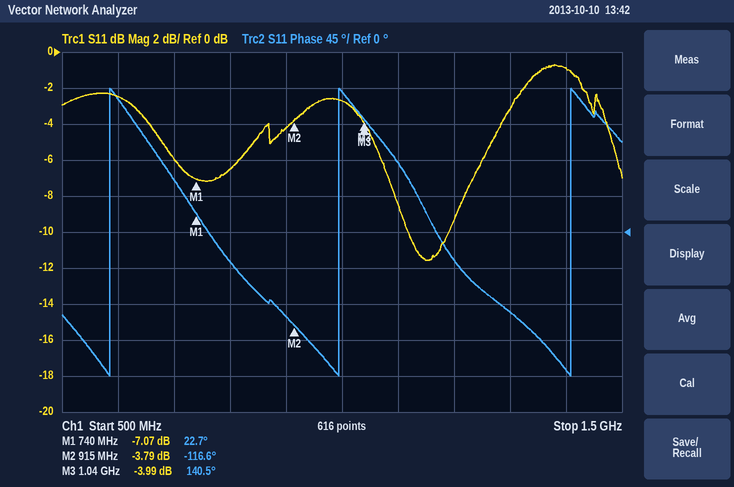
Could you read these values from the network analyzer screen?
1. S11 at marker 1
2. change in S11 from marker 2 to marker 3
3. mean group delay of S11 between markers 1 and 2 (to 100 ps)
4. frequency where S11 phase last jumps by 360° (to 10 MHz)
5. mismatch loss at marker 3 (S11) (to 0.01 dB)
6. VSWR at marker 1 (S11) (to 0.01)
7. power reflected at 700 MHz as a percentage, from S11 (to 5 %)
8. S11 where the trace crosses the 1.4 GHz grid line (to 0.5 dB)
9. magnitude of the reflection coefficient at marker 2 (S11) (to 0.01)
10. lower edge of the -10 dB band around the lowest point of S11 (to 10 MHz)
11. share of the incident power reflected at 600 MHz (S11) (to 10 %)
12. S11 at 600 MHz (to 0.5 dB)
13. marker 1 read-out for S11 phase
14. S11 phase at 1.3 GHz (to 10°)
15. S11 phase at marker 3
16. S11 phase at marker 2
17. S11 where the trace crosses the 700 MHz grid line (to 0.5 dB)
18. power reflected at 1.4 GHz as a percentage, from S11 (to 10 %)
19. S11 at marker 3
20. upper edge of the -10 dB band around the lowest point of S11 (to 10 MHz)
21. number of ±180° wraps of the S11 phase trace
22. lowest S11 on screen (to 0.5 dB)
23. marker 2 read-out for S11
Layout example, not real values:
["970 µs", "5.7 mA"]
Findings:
["-7.07 dB", "-0.20 dB", "2.2 ns", "1.41 GHz", "2.21 dB", "2.59", "25 %", "-1.0 dB", "0.65", "1.12 GHz", "60 %", "-2.5 dB", "22.7°", "-100°", "140.5°", "-116.6°", "-6.0 dB", "80 %", "-3.99 dB", "1.19 GHz", "3", "-11.5 dB", "-3.79 dB"]
